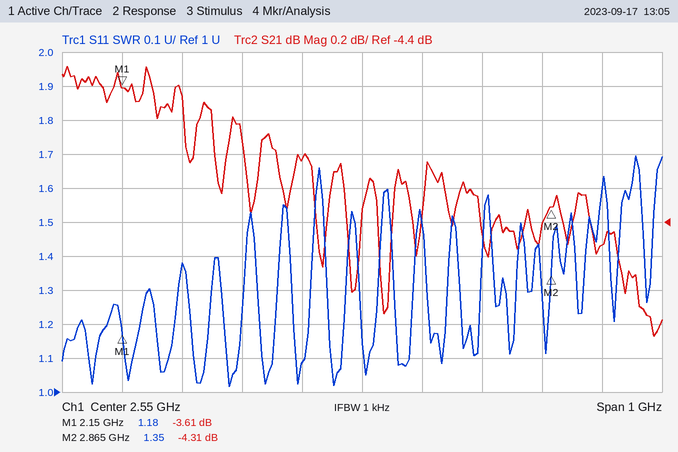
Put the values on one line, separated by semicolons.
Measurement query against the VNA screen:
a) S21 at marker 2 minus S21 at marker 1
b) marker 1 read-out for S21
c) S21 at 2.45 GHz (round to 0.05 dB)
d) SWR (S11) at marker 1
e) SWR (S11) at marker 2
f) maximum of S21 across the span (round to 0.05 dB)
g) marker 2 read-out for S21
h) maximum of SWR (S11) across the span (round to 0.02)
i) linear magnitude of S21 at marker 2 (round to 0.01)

-0.70 dB; -3.61 dB; -4.05 dB; 1.18; 1.35; -3.50 dB; -4.31 dB; 1.70; 0.61
